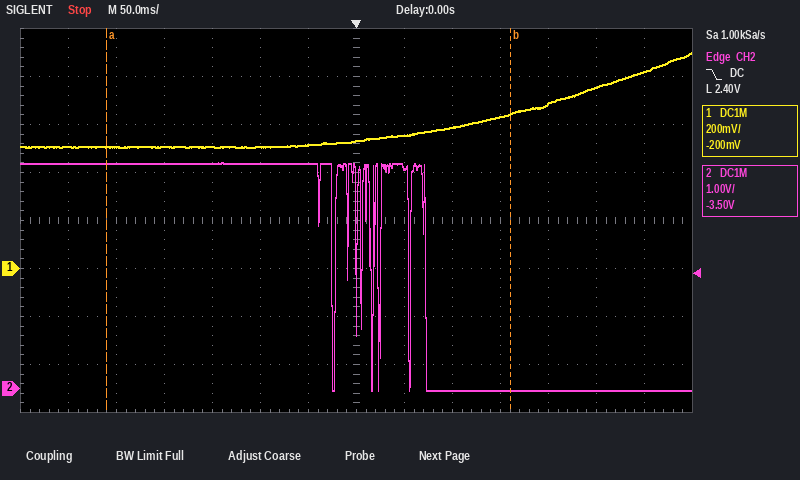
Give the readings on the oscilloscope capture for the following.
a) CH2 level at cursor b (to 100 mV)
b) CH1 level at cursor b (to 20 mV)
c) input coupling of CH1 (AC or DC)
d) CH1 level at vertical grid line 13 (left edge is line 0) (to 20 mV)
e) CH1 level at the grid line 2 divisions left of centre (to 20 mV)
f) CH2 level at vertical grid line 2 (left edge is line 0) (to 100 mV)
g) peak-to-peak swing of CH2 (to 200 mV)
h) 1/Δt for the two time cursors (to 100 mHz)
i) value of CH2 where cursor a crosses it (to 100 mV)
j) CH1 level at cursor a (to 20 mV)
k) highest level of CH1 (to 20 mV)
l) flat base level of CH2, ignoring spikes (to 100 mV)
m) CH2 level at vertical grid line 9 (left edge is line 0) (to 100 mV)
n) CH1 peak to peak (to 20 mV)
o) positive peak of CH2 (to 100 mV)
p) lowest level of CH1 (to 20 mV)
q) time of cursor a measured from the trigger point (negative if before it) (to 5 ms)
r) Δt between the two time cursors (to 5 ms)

0.0 V
640 mV
DC
820 mV
500 mV
4.7 V
4.8 V
2.4 Hz
4.7 V
500 mV
900 mV
0.0 V
0.0 V
400 mV
4.7 V
500 mV
-260 ms
420 ms
